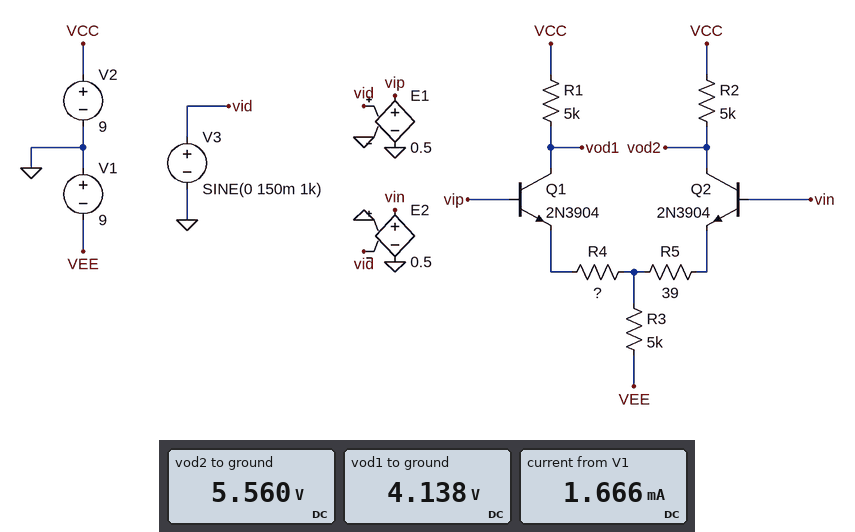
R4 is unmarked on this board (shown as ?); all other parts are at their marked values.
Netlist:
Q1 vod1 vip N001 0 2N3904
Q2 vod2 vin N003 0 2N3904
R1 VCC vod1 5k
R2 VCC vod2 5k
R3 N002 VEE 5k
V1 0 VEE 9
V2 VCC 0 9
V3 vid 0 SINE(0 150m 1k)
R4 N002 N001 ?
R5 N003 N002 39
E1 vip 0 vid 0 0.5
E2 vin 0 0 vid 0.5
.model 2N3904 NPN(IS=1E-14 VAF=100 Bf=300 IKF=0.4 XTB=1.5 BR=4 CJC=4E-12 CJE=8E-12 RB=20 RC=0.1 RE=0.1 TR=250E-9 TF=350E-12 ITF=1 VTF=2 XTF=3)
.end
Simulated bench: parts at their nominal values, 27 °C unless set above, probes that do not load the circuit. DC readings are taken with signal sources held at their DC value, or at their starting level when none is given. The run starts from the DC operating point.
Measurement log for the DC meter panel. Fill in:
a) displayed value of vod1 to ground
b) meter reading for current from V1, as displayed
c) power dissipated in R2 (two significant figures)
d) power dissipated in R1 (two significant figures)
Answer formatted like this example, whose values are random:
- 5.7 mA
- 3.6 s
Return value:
- 4.138 V
- 1.666 mA
- 2.4 mW
- 4.7 mW
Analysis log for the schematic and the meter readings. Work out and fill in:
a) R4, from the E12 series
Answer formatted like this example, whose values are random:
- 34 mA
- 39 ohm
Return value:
- 18 Ω
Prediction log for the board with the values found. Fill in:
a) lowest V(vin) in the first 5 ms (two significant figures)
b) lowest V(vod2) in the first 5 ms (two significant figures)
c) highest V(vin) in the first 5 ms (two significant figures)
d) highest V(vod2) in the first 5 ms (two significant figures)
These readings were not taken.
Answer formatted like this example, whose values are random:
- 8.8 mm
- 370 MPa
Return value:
- -75 mV
- 970 mV
- 75 mV
- 8.9 V
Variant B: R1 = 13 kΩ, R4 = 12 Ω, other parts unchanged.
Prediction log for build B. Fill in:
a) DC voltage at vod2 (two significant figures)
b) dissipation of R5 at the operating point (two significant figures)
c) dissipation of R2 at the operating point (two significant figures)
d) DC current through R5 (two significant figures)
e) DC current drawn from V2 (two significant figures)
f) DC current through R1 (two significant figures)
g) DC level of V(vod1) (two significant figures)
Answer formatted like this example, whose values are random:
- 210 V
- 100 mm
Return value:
- 5.1 V
- 24 µW
- 3.0 mW
- 780 µA
- 1.5 mA
- 740 µA
- -640 mV
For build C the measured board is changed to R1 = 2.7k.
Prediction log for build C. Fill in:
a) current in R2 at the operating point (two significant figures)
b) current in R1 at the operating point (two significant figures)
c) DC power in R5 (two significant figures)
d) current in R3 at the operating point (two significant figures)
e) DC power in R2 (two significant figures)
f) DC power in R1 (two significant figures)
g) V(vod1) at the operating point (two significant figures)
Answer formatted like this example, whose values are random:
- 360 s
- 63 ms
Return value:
- 680 µA
- 980 µA
- 18 µW
- 1.7 mA
- 2.3 mW
- 2.6 mW
- 6.4 V
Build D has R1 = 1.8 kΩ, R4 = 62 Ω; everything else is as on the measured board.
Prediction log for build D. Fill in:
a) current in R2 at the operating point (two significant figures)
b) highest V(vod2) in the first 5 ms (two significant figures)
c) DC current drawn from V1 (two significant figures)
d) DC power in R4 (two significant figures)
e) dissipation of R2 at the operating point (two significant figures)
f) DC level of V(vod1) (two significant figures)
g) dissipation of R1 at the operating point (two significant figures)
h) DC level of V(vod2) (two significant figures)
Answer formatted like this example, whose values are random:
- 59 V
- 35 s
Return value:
- 940 µA
- 8.3 V
- 1.7 mA
- 32 µW
- 4.4 mW
- 7.7 V
- 930 µW
- 4.3 V
